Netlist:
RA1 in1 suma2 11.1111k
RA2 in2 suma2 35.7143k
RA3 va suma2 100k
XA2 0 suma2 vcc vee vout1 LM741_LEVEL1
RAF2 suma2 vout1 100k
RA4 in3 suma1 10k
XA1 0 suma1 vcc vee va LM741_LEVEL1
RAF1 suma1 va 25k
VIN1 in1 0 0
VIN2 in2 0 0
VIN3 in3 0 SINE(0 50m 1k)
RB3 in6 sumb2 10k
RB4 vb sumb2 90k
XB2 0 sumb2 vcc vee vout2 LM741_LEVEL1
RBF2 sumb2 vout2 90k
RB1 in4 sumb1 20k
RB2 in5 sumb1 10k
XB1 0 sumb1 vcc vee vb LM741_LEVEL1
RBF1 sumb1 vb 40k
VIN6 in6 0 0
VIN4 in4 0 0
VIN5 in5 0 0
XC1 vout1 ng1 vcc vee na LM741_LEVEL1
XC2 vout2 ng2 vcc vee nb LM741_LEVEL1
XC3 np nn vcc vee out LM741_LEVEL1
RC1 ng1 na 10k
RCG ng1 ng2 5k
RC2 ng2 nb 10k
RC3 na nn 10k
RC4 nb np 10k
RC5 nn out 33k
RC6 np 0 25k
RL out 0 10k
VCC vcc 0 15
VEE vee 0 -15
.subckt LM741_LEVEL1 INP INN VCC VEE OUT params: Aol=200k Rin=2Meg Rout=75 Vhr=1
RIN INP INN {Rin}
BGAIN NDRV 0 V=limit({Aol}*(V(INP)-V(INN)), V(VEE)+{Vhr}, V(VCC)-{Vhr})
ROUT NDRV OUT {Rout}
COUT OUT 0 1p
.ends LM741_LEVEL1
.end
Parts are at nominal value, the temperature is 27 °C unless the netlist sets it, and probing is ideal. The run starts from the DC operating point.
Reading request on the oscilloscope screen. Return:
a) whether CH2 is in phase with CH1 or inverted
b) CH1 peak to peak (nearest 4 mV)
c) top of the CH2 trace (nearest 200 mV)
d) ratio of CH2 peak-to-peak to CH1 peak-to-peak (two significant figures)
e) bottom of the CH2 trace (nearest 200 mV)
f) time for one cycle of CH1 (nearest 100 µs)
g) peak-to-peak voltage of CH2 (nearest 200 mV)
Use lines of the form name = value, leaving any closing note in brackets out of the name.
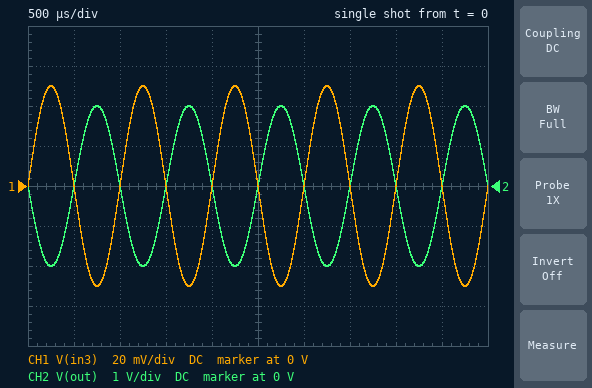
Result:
whether CH2 is in phase with CH1 or inverted = inverted
CH1 peak to peak = 100 mV
top of the CH2 trace = 2.0 V
ratio of CH2 peak-to-peak to CH1 peak-to-peak = 40
bottom of the CH2 trace = -2.0 V
time for one cycle of CH1 = 1.0 ms
peak-to-peak voltage of CH2 = 4.0 V
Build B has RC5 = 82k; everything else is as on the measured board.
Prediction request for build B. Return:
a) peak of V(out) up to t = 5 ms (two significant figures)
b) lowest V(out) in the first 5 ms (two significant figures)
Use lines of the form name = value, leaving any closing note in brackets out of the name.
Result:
peak of V(out) up to t = 5 ms = 4.7 V
lowest V(out) in the first 5 ms = -4.7 V
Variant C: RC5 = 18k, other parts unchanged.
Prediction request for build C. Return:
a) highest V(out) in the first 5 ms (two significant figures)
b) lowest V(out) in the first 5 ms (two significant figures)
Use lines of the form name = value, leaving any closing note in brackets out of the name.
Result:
highest V(out) in the first 5 ms = 1.2 V
lowest V(out) in the first 5 ms = -1.2 V
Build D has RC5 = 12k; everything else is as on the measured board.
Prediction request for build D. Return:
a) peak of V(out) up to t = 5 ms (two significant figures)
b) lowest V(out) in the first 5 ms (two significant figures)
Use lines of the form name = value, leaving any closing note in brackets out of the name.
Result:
peak of V(out) up to t = 5 ms = 840 mV
lowest V(out) in the first 5 ms = -840 mV
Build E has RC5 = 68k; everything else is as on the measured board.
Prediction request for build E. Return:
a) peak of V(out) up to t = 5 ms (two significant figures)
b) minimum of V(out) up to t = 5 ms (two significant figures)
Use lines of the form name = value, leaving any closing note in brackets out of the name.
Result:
peak of V(out) up to t = 5 ms = 3.9 V
minimum of V(out) up to t = 5 ms = -3.9 V
